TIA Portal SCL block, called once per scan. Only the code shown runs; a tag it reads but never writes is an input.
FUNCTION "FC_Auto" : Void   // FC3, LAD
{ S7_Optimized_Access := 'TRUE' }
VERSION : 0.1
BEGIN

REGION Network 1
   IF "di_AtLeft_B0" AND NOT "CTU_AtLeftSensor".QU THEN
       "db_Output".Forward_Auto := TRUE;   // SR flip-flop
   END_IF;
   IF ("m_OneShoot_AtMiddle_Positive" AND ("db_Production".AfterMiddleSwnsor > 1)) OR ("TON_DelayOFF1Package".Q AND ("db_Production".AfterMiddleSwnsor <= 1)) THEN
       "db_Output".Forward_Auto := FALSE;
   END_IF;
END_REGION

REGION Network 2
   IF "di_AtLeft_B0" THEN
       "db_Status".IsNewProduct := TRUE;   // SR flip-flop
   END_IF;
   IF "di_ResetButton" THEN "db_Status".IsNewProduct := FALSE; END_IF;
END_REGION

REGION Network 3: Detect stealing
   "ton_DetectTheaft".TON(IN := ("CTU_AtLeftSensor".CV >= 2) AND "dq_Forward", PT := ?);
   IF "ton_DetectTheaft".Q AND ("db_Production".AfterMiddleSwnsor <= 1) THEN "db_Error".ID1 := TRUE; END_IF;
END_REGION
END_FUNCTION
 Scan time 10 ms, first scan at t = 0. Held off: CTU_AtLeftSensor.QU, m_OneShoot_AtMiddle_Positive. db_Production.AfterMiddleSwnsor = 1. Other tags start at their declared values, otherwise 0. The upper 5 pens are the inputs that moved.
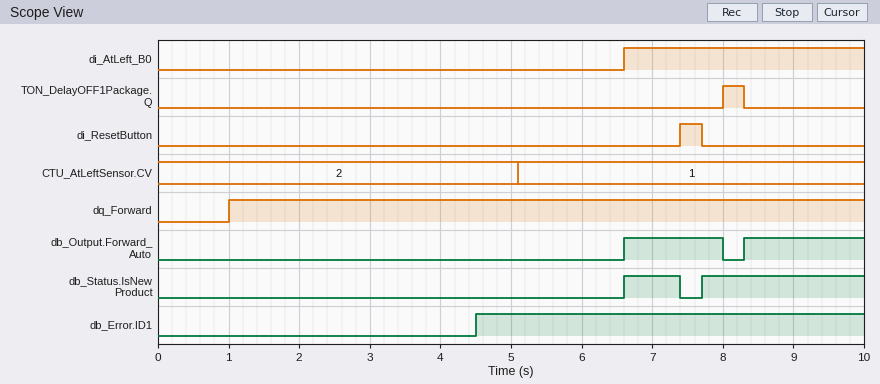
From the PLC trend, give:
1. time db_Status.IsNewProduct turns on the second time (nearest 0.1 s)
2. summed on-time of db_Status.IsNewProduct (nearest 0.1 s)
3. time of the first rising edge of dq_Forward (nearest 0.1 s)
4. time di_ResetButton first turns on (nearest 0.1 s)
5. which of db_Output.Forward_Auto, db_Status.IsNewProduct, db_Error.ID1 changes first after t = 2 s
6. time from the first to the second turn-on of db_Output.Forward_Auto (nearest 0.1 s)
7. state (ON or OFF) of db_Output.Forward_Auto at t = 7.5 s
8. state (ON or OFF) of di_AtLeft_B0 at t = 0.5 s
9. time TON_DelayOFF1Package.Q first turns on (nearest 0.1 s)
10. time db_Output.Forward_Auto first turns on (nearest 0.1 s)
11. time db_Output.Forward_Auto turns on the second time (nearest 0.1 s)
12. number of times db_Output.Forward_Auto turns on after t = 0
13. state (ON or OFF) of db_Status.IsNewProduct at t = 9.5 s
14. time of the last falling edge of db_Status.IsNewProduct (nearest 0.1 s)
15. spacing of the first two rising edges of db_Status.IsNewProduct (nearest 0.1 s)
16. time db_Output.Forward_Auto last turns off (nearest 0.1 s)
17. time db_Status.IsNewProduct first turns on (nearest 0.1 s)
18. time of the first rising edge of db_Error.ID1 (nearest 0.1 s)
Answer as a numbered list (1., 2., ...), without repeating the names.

1. 7.7 s
2. 3.1 s
3. 1.0 s
4. 7.4 s
5. db_Error.ID1
6. 1.7 s
7. ON
8. OFF
9. 8.0 s
10. 6.6 s
11. 8.3 s
12. 2
13. ON
14. 7.4 s
15. 1.1 s
16. 8.0 s
17. 6.6 s
18. 4.5 s
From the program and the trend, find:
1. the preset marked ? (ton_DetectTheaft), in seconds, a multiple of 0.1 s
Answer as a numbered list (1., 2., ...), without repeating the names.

1. 3.5 s
